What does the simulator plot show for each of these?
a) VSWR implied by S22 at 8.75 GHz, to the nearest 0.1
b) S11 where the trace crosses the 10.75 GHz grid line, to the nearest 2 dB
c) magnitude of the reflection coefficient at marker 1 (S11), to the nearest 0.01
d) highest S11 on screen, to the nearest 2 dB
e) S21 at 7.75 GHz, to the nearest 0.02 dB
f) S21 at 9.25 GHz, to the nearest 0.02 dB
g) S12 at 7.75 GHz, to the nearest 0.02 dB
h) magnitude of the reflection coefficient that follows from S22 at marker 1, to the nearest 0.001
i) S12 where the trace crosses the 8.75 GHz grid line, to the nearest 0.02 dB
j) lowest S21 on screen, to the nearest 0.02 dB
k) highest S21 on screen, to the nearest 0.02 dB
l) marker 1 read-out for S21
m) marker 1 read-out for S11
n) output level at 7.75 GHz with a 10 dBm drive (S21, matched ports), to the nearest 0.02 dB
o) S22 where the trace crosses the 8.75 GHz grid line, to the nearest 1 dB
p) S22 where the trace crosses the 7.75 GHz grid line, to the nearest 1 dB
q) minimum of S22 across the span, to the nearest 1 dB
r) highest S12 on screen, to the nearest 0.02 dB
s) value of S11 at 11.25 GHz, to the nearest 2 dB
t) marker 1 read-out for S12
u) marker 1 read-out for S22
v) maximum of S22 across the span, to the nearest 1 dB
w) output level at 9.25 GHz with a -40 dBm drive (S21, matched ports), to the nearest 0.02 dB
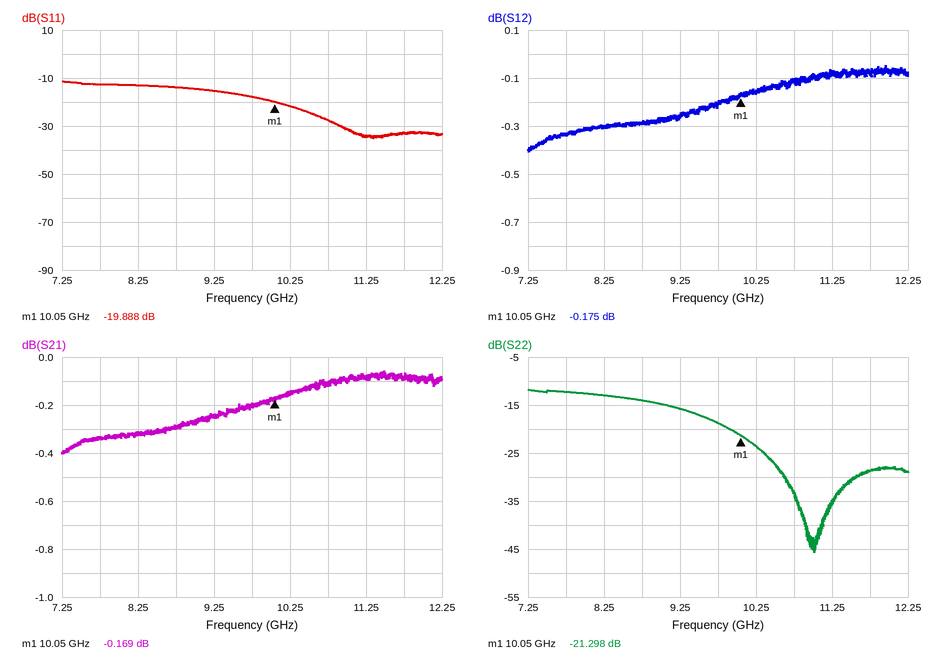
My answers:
1.5
-28 dB
0.10
-12 dB
-0.34 dB
-0.24 dB
-0.34 dB
0.086
-0.28 dB
-0.40 dB
-0.06 dB
-0.169 dB
-19.888 dB
9.66 dBm
-14 dB
-12 dB
-46 dB
-0.04 dB
-34 dB
-0.175 dB
-21.298 dB
-12 dB
-40.24 dBm
